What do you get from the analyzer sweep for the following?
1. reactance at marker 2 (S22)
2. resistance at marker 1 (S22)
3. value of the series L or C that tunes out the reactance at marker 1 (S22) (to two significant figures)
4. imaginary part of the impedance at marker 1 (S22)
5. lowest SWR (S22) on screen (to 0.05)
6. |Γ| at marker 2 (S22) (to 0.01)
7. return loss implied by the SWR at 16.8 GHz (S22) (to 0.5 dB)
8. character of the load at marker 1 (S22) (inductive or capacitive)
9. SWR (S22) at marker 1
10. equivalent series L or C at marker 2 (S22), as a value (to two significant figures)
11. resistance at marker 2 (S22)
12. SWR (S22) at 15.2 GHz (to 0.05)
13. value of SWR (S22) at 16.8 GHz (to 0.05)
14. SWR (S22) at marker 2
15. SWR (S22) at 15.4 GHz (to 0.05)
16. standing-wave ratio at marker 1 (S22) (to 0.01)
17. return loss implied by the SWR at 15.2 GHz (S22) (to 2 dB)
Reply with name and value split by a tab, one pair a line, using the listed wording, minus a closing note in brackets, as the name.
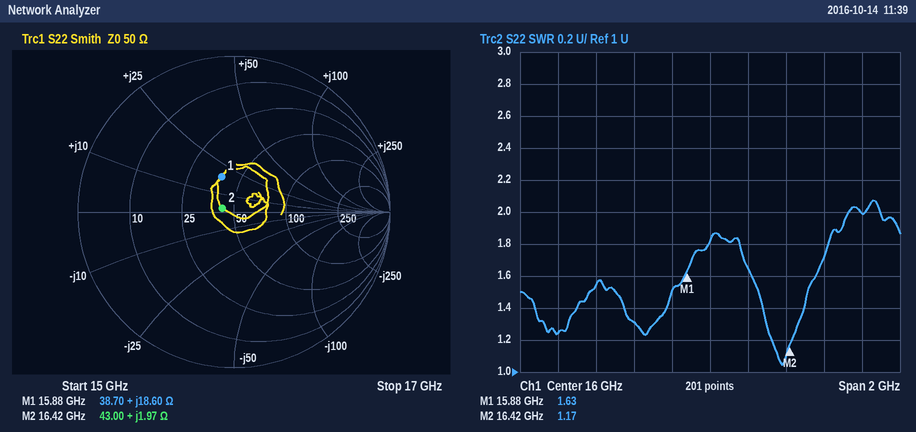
reactance at marker 2	+1.97 Ω
resistance at marker 1	38.70 Ω
value of the series L or C that tunes out the reactance at marker 1 (S22)	540 fF
imaginary part of the impedance at marker 1	+18.60 Ω
lowest SWR (S22) on screen	1.05
|Γ| at marker 2 (S22)	0.08
return loss implied by the SWR at 16.8 GHz (S22)	9.5 dB
character of the load at marker 1 (S22)	inductive
SWR (S22) at marker 1	1.63
equivalent series L or C at marker 2 (S22), as a value	19 pH
resistance at marker 2	43.00 Ω
SWR (S22) at 15.2 GHz	1.25
value of SWR (S22) at 16.8 GHz	2.00
SWR (S22) at marker 2	1.17
SWR (S22) at 15.4 GHz	1.55
standing-wave ratio at marker 1 (S22)	1.63
return loss implied by the SWR at 15.2 GHz (S22)	20 dB
